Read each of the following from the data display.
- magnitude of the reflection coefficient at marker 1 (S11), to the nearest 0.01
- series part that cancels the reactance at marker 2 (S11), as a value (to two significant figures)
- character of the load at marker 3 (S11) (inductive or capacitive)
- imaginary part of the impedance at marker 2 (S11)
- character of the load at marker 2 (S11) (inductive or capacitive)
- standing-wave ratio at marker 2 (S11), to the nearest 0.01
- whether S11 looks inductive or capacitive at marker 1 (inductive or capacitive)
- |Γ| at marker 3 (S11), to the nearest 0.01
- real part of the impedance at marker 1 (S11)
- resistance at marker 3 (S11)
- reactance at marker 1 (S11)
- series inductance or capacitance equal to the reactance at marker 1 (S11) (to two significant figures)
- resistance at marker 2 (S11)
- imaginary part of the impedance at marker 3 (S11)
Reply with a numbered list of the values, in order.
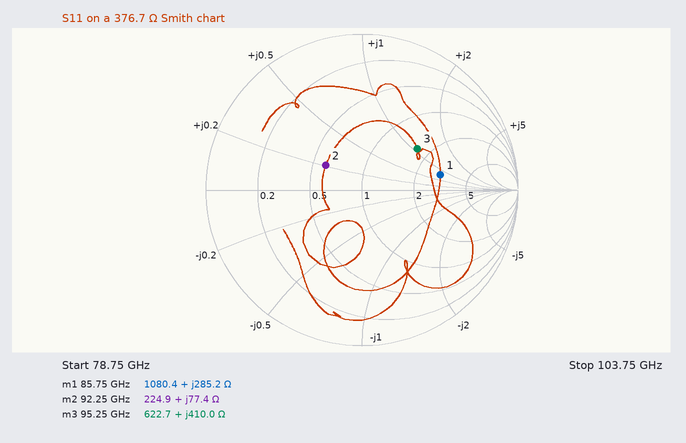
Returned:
1. 0.51
2. 22 fF
3. inductive
4. +77.4 Ω
5. inductive
6. 1.78
7. inductive
8. 0.44
9. 1080.4 Ω
10. 622.7 Ω
11. +285.2 Ω
12. 530 pH
13. 224.9 Ω
14. +410.0 Ω
